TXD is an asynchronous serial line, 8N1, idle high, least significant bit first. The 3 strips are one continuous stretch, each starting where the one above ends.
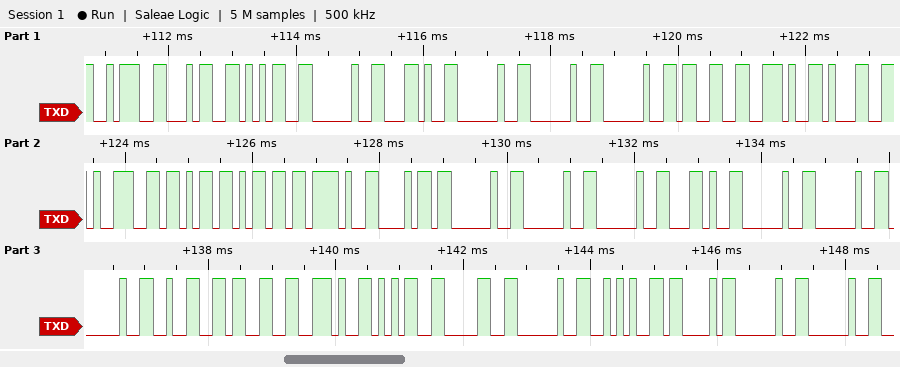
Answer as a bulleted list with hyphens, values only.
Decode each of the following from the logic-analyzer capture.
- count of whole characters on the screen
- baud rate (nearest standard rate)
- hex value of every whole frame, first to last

- 33
- 9600 baud
- 0x3A 0x34 0x35 0x20 0x2C 0x20 0x20 0x20 0x33 0x2E 0x31 0x39 0x6B 0x6D 0x2F 0x68 0x20 0x20 0x20 0x2C 0x20 0x20 0x20 0x32 0x33 0x2E 0x35 0x30 0x20 0x2A 0x43 0x20 0x20
